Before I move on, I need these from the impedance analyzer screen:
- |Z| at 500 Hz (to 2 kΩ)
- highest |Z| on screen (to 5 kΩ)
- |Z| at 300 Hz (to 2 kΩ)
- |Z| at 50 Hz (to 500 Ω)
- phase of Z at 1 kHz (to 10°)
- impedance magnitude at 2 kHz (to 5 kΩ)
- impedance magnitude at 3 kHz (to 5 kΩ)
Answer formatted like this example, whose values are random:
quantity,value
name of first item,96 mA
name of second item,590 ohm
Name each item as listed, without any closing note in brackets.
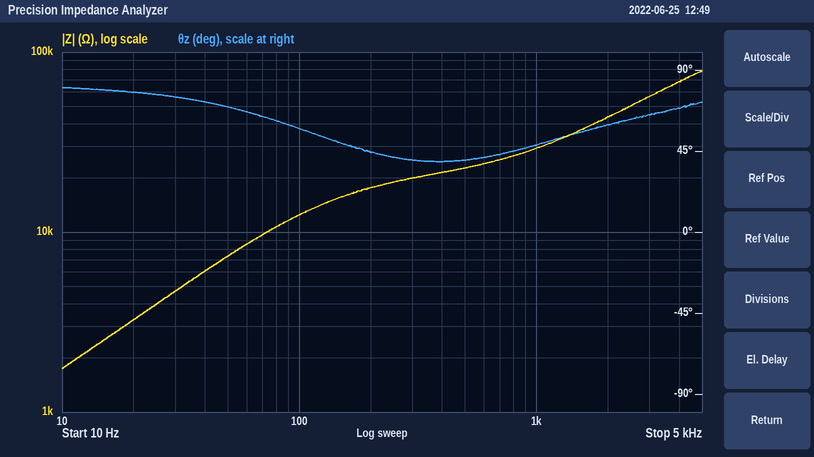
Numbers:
quantity,value
|Z| at 500 Hz,22 kΩ
highest |Z| on screen,80 kΩ
|Z| at 300 Hz,20 kΩ
|Z| at 50 Hz,7.5 kΩ
phase of Z at 1 kHz,50°
impedance magnitude at 2 kHz,45 kΩ
impedance magnitude at 3 kHz,55 kΩ
